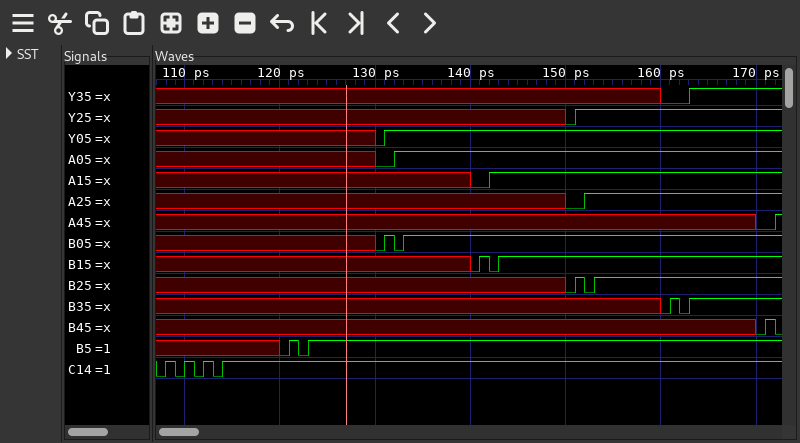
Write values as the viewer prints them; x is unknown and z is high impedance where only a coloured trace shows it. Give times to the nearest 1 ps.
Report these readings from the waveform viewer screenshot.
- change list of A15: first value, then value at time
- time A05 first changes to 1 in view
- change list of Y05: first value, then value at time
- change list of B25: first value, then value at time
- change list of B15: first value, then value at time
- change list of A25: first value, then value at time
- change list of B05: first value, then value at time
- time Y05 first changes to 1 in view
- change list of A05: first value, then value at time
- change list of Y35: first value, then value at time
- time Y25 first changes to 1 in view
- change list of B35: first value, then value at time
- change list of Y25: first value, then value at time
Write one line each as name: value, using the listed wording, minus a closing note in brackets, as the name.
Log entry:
change list of A15: first value, then value at time: x, 0 at 140 ps, 1 at 142 ps
time A05 first changes to 1 in view: 132 ps
change list of Y05: first value, then value at time: x, 0 at 130 ps, 1 at 131 ps
change list of B25: first value, then value at time: x, 0 at 150 ps, 1 at 151 ps, 0 at 152 ps, 1 at 153 ps
change list of B15: first value, then value at time: x, 0 at 140 ps, 1 at 141 ps, 0 at 142 ps, 1 at 143 ps
change list of A25: first value, then value at time: x, 0 at 150 ps, 1 at 152 ps
change list of B05: first value, then value at time: x, 0 at 130 ps, 1 at 131 ps, 0 at 132 ps, 1 at 133 ps
time Y05 first changes to 1 in view: 131 ps
change list of A05: first value, then value at time: x, 0 at 130 ps, 1 at 132 ps
change list of Y35: first value, then value at time: x, 0 at 160 ps, 1 at 163 ps
time Y25 first changes to 1 in view: 151 ps
change list of B35: first value, then value at time: x, 0 at 160 ps, 1 at 161 ps, 0 at 162 ps, 1 at 163 ps
change list of Y25: first value, then value at time: x, 0 at 150 ps, 1 at 151 ps
